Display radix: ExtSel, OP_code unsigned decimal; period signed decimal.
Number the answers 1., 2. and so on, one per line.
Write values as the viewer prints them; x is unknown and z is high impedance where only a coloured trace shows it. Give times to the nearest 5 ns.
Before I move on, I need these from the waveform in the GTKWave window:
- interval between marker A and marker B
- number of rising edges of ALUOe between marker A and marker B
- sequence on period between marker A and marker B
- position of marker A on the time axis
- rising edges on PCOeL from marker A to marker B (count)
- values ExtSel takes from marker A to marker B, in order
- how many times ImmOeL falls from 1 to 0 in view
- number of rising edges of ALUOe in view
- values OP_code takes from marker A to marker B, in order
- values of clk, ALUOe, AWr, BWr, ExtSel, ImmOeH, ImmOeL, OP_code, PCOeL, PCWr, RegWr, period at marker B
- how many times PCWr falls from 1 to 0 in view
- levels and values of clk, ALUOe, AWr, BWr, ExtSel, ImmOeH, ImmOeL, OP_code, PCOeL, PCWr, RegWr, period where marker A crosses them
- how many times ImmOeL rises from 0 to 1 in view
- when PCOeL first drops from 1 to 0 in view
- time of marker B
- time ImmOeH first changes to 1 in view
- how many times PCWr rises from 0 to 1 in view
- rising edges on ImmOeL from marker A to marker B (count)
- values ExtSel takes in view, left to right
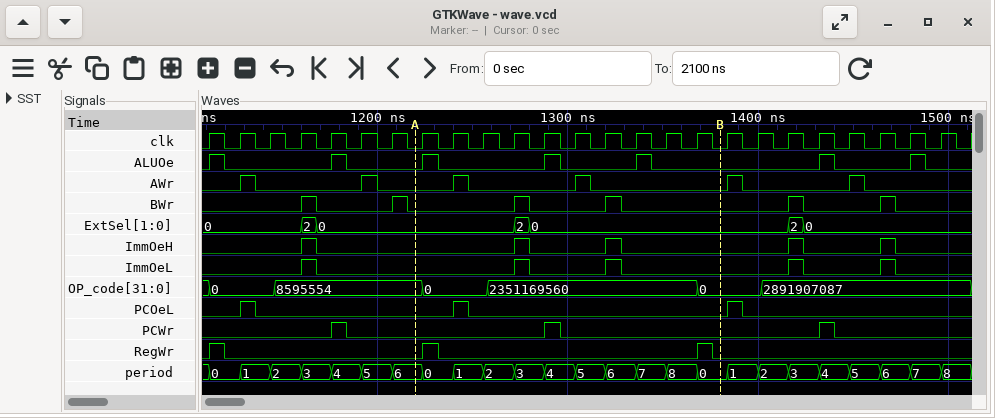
1. 160 ns
2. 3
3. 6, 0, 1, 2, 3, 4, 5, 6, 7, 8, 0
4. 1220 ns
5. 1
6. 0, 2, 0
7. 5
8. 7
9. 8595554, 0, 2351169560, 0
10. clk=0, ALUOe=0, AWr=0, BWr=0, ExtSel=0, ImmOeH=0, ImmOeL=0, OP_code=0, PCOeL=0, PCWr=0, RegWr=0, period=0
11. 3
12. clk=0, ALUOe=0, AWr=0, BWr=0, ExtSel=0, ImmOeH=0, ImmOeL=0, OP_code=8595554, PCOeL=0, PCWr=0, RegWr=0, period=6
13. 5
14. 1135 ns
15. 1380 ns
16. 1160 ns
17. 3
18. 2
19. 0, 2, 0, 2, 0, 2, 0
